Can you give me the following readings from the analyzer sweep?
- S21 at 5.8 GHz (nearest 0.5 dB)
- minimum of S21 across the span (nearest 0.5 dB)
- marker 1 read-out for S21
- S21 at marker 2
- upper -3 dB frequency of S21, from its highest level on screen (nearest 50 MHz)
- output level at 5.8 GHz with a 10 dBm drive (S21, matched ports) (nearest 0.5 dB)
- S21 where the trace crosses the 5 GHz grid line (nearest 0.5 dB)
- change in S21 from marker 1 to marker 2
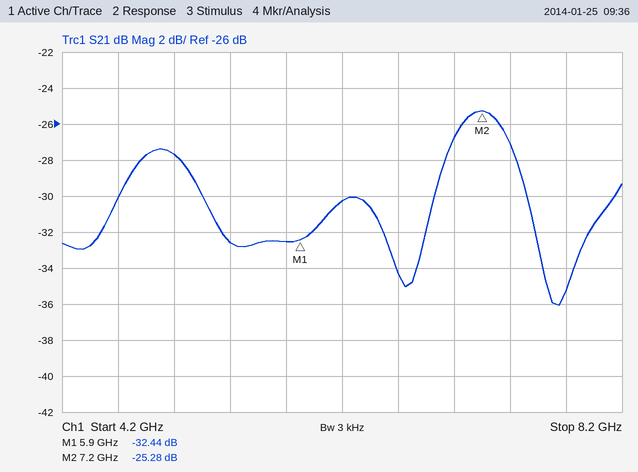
-32.5 dB
-36.0 dB
-32.44 dB
-25.28 dB
7.45 GHz
-22.5 dBm
-27.5 dB
7.16 dB
